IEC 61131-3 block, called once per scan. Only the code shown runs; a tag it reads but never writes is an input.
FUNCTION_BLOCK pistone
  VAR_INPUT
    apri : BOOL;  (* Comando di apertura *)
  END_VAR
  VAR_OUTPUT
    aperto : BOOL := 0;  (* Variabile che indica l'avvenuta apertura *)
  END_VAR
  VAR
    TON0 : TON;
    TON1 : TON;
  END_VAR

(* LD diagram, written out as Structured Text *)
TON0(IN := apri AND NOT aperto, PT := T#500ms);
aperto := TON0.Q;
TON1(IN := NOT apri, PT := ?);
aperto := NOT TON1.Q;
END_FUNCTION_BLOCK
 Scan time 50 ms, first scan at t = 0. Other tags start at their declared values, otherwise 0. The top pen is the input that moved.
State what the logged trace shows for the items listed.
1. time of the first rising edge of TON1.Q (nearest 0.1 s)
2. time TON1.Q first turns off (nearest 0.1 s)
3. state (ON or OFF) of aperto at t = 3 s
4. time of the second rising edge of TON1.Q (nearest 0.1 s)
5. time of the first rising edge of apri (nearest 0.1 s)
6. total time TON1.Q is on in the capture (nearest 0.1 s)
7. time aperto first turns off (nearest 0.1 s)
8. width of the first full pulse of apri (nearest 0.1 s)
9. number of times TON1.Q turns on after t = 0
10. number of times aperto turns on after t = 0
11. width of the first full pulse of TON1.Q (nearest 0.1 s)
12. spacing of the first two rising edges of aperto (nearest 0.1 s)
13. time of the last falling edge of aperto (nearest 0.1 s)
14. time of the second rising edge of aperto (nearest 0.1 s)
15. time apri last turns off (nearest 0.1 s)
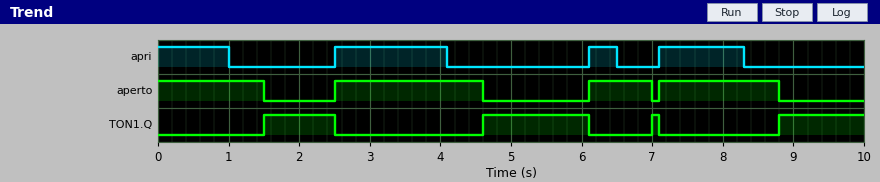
1.5 s
2.5 s
ON
4.6 s
2.5 s
3.8 s
1.5 s
1.6 s
4
3
1.0 s
3.6 s
8.8 s
6.1 s
8.3 s
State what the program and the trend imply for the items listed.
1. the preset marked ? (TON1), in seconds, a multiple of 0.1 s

0.5 s
